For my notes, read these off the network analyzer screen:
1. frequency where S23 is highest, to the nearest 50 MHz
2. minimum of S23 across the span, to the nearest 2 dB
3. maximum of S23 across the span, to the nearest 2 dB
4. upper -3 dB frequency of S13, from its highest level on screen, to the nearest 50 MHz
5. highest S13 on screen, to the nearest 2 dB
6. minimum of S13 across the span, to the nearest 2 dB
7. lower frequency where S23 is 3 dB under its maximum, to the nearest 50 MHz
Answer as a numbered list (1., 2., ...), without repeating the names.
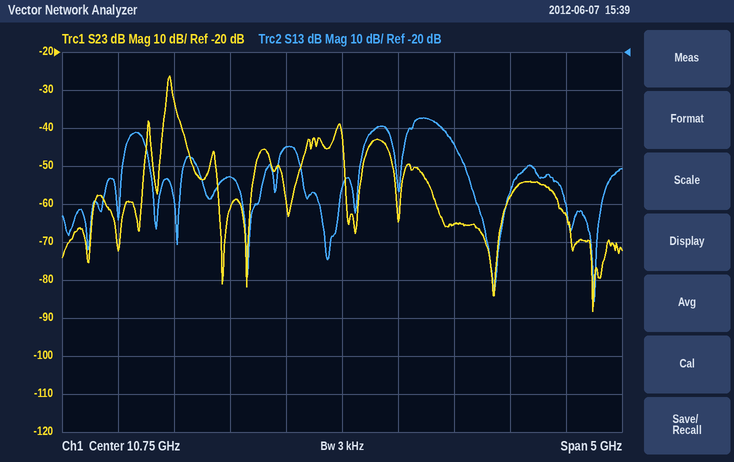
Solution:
1. 9.20 GHz
2. -88 dB
3. -26 dB
4. 11.65 GHz
5. -38 dB
6. -86 dB
7. 9.20 GHz
